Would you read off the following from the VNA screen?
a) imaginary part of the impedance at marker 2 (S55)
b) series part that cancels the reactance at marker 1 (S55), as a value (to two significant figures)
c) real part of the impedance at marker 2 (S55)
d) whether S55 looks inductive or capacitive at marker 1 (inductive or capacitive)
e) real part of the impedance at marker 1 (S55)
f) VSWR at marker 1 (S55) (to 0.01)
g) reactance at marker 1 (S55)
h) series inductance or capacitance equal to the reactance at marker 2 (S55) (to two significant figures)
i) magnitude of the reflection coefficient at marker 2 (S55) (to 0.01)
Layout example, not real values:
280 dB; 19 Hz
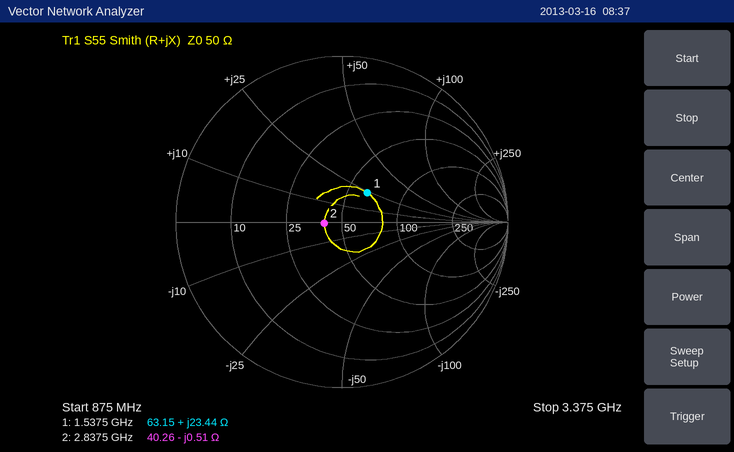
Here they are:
-0.51 Ω; 4.4 pF; 40.26 Ω; inductive; 63.15 Ω; 1.61; +23.44 Ω; 110 pF; 0.11
